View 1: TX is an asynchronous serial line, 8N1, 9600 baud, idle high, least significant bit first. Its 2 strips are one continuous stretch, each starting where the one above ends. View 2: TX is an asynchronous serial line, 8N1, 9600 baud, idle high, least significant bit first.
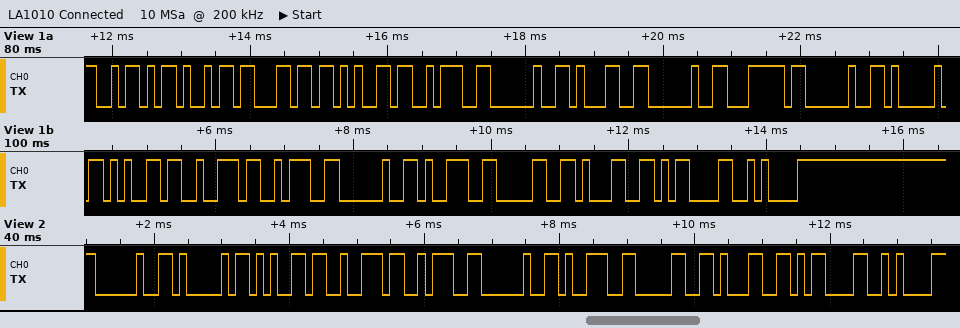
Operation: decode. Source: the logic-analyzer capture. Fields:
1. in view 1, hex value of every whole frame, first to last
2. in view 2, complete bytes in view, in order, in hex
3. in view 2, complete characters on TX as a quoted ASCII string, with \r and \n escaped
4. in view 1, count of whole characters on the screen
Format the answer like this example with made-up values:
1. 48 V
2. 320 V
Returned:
1. 5A 69 6C 65 3A 20 31 20 7C 20 41 65 72 3A 20 39 30 31 0D 0A
2. 20 41 65 72 3A 20 39 30 31 0D 0A
3. " Aer: 901\r\n"
4. 20
